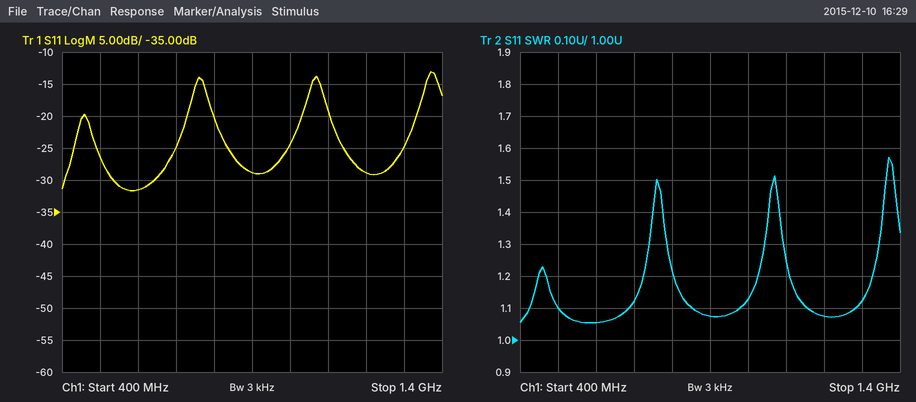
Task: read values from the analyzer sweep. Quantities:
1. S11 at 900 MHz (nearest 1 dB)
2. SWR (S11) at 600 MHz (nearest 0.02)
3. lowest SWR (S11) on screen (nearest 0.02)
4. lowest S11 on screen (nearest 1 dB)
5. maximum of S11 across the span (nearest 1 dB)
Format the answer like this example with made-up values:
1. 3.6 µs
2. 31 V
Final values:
1. -29 dB
2. 1.06
3. 1.06
4. -32 dB
5. -13 dB
